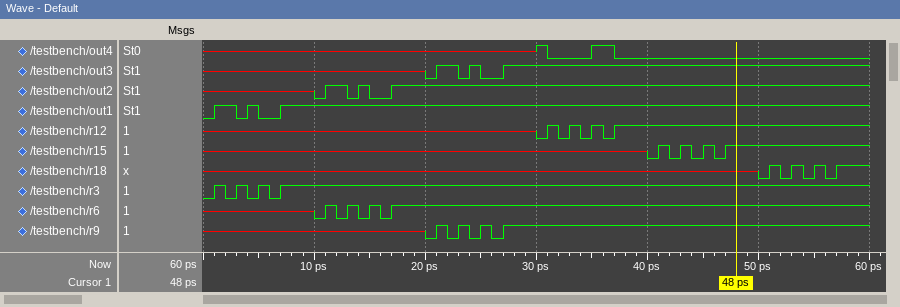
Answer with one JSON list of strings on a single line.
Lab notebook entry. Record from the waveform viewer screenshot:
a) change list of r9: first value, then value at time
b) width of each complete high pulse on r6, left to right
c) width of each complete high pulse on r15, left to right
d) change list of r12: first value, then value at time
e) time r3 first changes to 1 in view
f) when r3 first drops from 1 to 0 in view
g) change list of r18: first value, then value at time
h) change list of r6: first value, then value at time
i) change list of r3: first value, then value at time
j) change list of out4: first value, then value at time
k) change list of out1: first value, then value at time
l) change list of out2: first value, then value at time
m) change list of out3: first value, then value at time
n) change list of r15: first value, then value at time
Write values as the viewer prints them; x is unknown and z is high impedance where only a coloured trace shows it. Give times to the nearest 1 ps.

["x, 0 at 20 ps, 1 at 21 ps, 0 at 22 ps, 1 at 23 ps, 0 at 24 ps, 1 at 25 ps, 0 at 26 ps, 1 at 27 ps", "1 ps, 1 ps, 1 ps", "1 ps, 1 ps, 1 ps", "x, 0 at 30 ps, 1 at 31 ps, 0 at 32 ps, 1 at 33 ps, 0 at 34 ps, 1 at 35 ps, 0 at 36 ps, 1 at 37 ps", "1 ps", "2 ps", "x, 0 at 50 ps, 1 at 51 ps, 0 at 52 ps, 1 at 53 ps, 0 at 54 ps, 1 at 55 ps, 0 at 56 ps, 1 at 57 ps", "x, 0 at 10 ps, 1 at 11 ps, 0 at 12 ps, 1 at 13 ps, 0 at 14 ps, 1 at 15 ps, 0 at 16 ps, 1 at 17 ps", "0, 1 at 1 ps, 0 at 2 ps, 1 at 3 ps, 0 at 4 ps, 1 at 5 ps, 0 at 6 ps, 1 at 7 ps", "x, 1 at 30 ps, 0 at 31 ps, 1 at 35 ps, 0 at 37 ps", "0, 1 at 1 ps, 0 at 3 ps, 1 at 4 ps, 0 at 5 ps, 1 at 7 ps", "x, 0 at 10 ps, 1 at 11 ps, 0 at 13 ps, 1 at 14 ps, 0 at 15 ps, 1 at 17 ps", "x, 0 at 20 ps, 1 at 21 ps, 0 at 23 ps, 1 at 24 ps, 0 at 25 ps, 1 at 27 ps", "x, 0 at 40 ps, 1 at 41 ps, 0 at 42 ps, 1 at 43 ps, 0 at 44 ps, 1 at 45 ps, 0 at 46 ps, 1 at 47 ps"]
